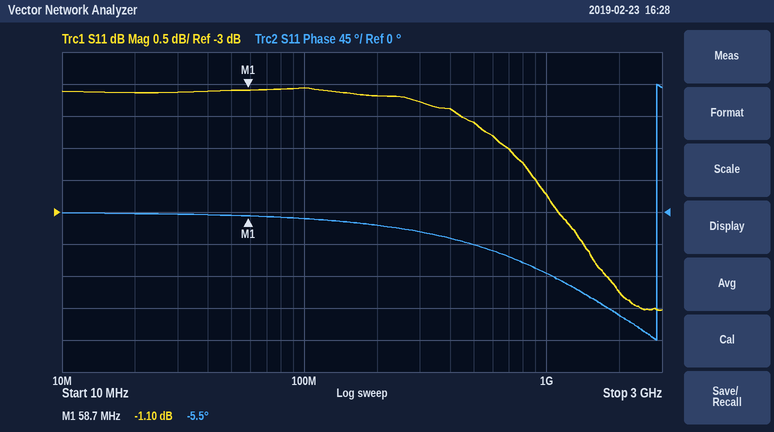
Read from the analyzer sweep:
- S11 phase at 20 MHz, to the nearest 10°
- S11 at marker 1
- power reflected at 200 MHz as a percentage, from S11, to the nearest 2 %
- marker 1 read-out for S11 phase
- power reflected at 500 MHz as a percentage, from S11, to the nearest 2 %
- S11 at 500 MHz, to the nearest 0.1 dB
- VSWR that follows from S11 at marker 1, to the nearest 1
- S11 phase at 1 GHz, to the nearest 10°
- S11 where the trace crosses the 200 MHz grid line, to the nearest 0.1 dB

0°
-1.10 dB
76 %
-5.5°
70 %
-1.6 dB
16
-90°
-1.2 dB
